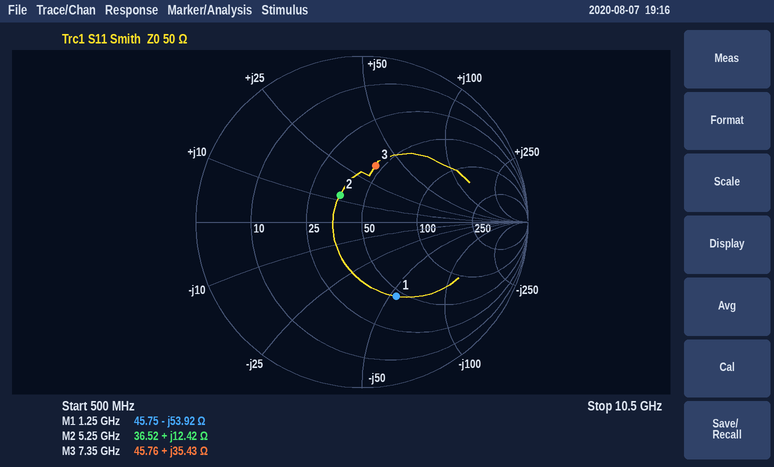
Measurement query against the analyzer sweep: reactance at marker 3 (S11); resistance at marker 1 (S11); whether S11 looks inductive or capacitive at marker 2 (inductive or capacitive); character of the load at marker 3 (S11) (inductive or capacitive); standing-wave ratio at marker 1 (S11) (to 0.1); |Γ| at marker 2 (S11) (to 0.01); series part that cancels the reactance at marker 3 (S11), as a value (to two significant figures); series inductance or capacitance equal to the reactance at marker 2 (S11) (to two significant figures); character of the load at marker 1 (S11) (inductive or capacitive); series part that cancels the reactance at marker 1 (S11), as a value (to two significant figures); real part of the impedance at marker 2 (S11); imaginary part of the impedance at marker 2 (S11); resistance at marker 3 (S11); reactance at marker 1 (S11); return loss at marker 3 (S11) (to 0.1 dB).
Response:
+35.43 Ω
45.75 Ω
inductive
inductive
2.9
0.21
610 fF
380 pH
capacitive
6.9 nH
36.52 Ω
+12.42 Ω
45.76 Ω
-53.92 Ω
9.1 dB
